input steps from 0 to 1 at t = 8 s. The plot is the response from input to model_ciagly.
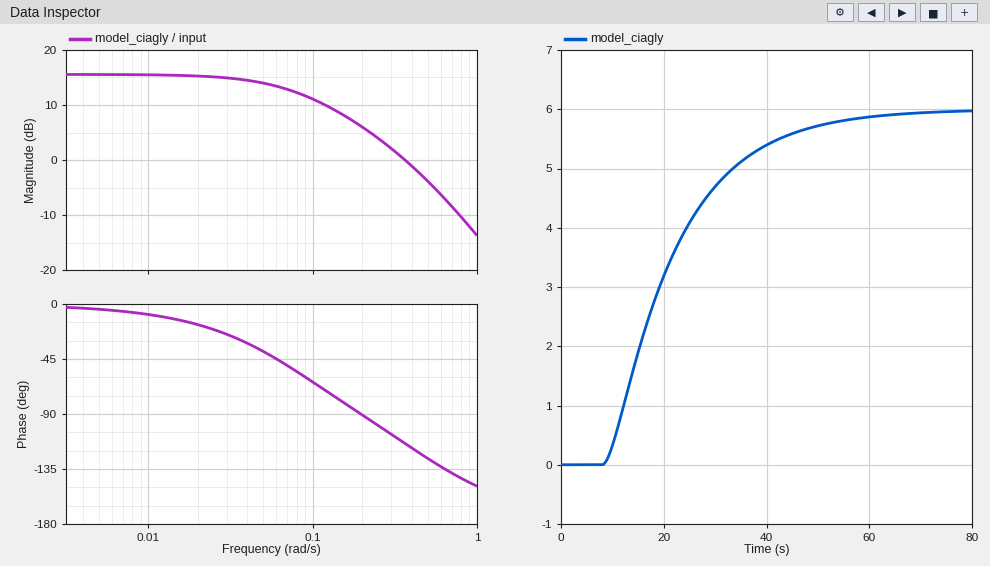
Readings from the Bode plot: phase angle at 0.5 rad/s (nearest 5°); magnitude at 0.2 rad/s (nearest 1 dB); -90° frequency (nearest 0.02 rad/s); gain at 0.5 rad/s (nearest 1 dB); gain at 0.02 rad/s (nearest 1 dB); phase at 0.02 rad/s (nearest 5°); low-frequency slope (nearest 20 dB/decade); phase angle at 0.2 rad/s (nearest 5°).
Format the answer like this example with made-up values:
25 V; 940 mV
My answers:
-125°; 6 dB; 0.20 rad/s; -4 dB; 15 dB; -15°; 0 dB/decade; -90°
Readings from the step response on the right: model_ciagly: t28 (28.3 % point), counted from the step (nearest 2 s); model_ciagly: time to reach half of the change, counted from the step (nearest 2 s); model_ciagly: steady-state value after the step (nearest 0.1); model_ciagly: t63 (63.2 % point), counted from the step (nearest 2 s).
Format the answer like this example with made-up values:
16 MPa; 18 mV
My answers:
6 s; 12 s; 6.0; 16 s
